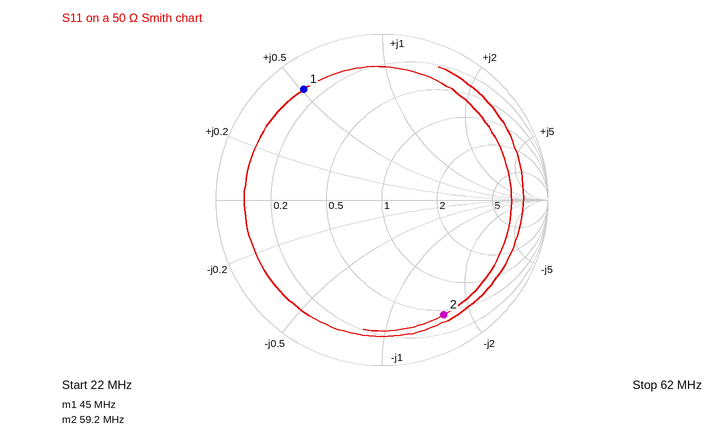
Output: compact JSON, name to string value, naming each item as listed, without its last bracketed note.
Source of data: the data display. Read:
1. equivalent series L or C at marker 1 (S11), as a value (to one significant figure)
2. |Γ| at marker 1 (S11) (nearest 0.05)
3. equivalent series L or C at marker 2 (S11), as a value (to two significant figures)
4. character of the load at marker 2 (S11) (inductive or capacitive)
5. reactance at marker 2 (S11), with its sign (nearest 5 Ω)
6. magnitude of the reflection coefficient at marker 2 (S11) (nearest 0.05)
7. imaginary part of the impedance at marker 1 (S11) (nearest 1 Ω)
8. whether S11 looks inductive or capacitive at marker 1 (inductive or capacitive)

{"equivalent series L or C at marker 1 (S11), as a value": "90 nH", "|Γ| at marker 1 (S11)": "0.80", "equivalent series L or C at marker 2 (S11), as a value": "34 pF", "character of the load at marker 2 (S11)": "capacitive", "reactance at marker 2 (S11), with its sign": "-80 Ω", "magnitude of the reflection coefficient at marker 2 (S11)": "0.80", "imaginary part of the impedance at marker 1 (S11)": "+26 Ω", "whether S11 looks inductive or capacitive at marker 1": "inductive"}
